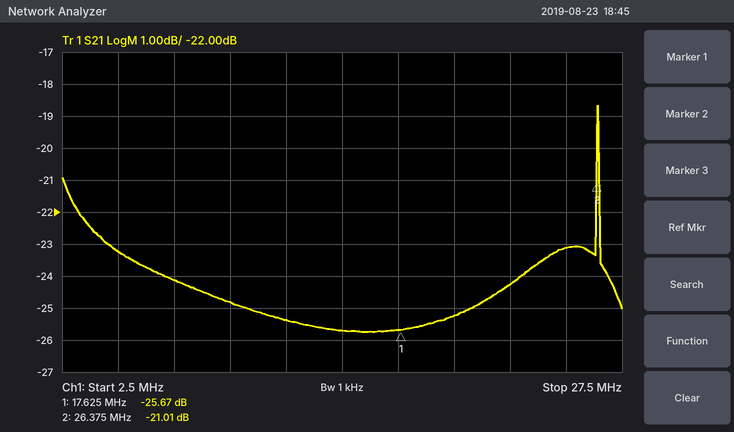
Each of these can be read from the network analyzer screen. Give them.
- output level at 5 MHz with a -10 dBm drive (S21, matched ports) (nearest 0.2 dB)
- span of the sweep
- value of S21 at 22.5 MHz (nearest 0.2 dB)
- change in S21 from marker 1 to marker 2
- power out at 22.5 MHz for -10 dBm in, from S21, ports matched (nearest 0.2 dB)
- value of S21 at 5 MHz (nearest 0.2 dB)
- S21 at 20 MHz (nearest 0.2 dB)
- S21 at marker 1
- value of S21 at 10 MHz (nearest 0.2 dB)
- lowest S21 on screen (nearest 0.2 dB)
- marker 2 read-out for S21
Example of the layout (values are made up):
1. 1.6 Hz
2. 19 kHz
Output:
1. -33.2 dBm
2. 25 MHz
3. -24.2 dB
4. 4.66 dB
5. -34.2 dBm
6. -23.2 dB
7. -25.2 dB
8. -25.67 dB
9. -24.8 dB
10. -25.8 dB
11. -21.01 dB
